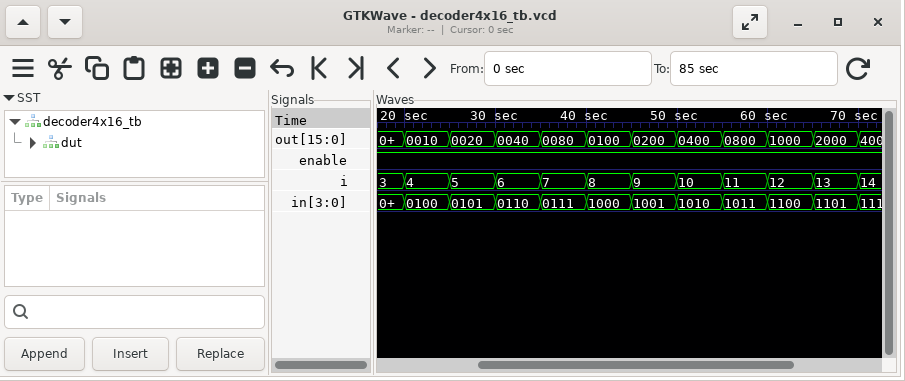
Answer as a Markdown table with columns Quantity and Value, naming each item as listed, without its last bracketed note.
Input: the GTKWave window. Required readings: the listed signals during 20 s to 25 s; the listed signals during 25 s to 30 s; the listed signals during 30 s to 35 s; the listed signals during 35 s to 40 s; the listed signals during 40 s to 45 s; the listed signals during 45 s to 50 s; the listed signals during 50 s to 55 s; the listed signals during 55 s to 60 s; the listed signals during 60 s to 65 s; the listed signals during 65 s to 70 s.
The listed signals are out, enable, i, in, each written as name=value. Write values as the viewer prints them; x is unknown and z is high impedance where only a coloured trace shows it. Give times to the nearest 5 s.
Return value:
| Quantity | Value |
|---|---|
| the listed signals during 20 s to 25 s | out=0010, enable=1, i=4, in=0100 |
| the listed signals during 25 s to 30 s | out=0020, enable=1, i=5, in=0101 |
| the listed signals during 30 s to 35 s | out=0040, enable=1, i=6, in=0110 |
| the listed signals during 35 s to 40 s | out=0080, enable=1, i=7, in=0111 |
| the listed signals during 40 s to 45 s | out=0100, enable=1, i=8, in=1000 |
| the listed signals during 45 s to 50 s | out=0200, enable=1, i=9, in=1001 |
| the listed signals during 50 s to 55 s | out=0400, enable=1, i=10, in=1010 |
| the listed signals during 55 s to 60 s | out=0800, enable=1, i=11, in=1011 |
| the listed signals during 60 s to 65 s | out=1000, enable=1, i=12, in=1100 |
| the listed signals during 65 s to 70 s | out=2000, enable=1, i=13, in=1101 |
